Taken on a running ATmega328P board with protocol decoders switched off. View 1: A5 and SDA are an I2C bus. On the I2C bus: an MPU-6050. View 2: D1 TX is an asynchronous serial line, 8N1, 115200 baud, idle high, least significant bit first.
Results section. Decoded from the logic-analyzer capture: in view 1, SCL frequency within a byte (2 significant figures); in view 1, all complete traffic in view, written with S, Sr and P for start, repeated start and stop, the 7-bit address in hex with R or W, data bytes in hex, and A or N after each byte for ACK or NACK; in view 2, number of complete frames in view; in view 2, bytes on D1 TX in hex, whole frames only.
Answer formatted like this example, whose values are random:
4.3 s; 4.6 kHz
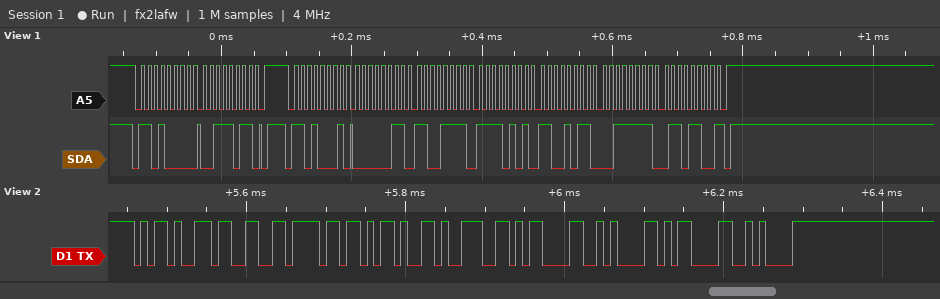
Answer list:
100 kHz; S 68W A 3B A P S 68R A 03 A CF A F5 A CB A 3F A 6C N P; 9; 2D 33 6F 2D 39 0D 0A 0D 0A
